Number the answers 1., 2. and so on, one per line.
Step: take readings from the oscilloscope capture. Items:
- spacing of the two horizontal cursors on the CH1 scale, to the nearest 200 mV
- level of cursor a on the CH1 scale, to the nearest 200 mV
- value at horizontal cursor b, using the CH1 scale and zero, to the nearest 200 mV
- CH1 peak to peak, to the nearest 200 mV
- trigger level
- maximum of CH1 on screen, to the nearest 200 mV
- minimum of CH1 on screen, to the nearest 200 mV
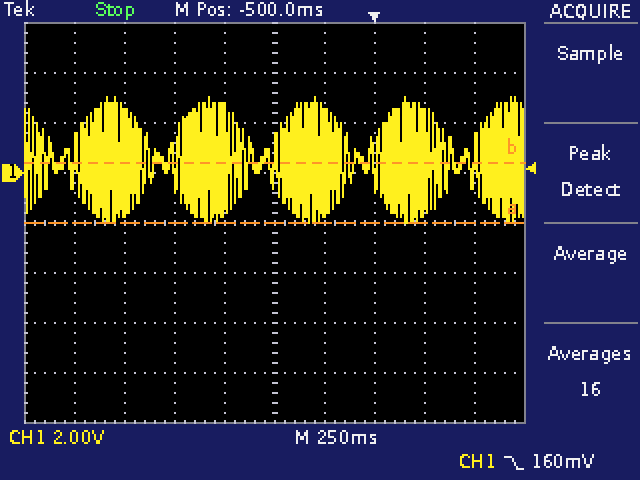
1. 2.4 V
2. -2.0 V
3. 400 mV
4. 5.0 V
5. 160 mV
6. 3.0 V
7. -2.0 V
